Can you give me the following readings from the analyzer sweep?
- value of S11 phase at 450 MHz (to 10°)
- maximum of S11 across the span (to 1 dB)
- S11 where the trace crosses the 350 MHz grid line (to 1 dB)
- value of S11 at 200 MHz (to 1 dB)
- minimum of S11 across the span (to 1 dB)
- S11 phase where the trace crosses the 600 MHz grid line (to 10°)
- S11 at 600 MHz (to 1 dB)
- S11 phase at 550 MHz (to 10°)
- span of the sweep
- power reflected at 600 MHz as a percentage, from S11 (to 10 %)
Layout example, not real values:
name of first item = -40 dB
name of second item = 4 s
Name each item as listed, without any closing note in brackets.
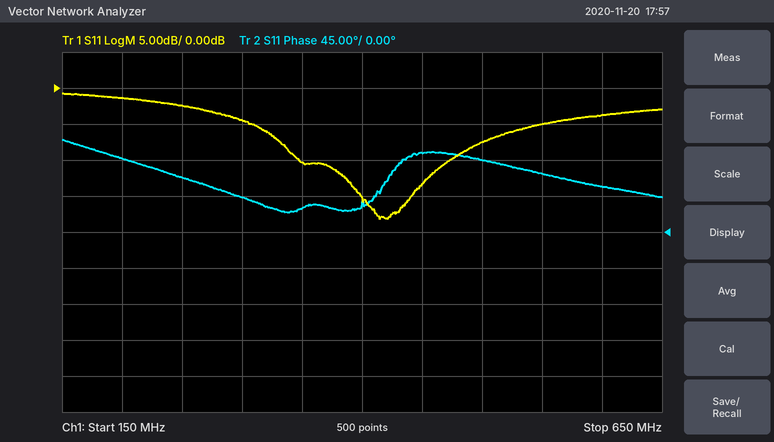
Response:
value of S11 phase at 450 MHz = 100°
maximum of S11 across the span = -1 dB
S11 where the trace crosses the 350 MHz grid line = -10 dB
value of S11 at 200 MHz = -1 dB
minimum of S11 across the span = -18 dB
S11 phase where the trace crosses the 600 MHz grid line = 60°
S11 at 600 MHz = -4 dB
S11 phase at 550 MHz = 70°
span of the sweep = 500 MHz
power reflected at 600 MHz as a percentage, from S11 = 40 %
